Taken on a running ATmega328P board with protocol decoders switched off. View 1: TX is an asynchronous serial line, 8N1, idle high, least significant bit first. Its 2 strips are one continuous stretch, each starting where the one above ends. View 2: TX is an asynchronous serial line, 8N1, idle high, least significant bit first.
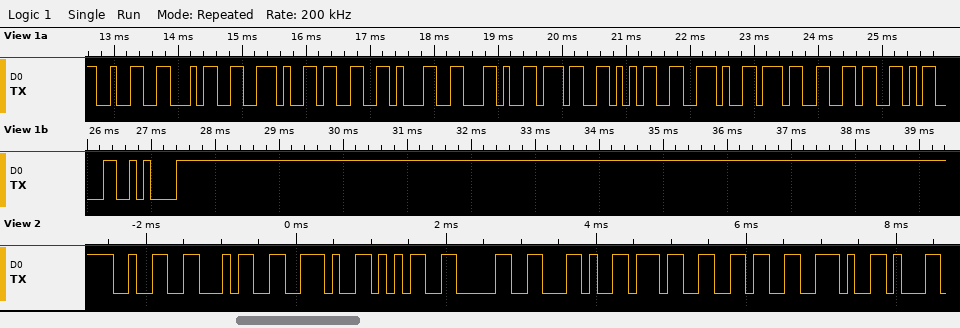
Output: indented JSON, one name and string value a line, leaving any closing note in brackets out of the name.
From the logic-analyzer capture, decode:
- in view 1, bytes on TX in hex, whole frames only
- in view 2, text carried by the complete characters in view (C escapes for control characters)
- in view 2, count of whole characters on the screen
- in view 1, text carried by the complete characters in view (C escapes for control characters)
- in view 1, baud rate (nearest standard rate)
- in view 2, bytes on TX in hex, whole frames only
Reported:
{
  "in view 1, bytes on TX in hex, whole frames only": "32 34 2E 33 31 2C 37 35 2E 37 36 0D 0A",
  "in view 2, text carried by the complete characters in view": "\"24.50,76.\"",
  "in view 2, count of whole characters on the screen": "9",
  "in view 1, text carried by the complete characters in view": "\"24.31,75.76\\r\\n\"",
  "in view 1, baud rate": "9600 baud",
  "in view 2, bytes on TX in hex, whole frames only": "32 34 2E 35 30 2C 37 36 2E"
}
